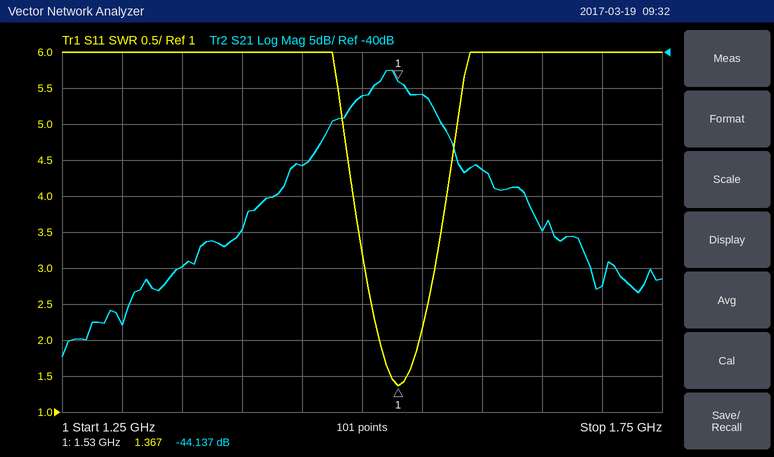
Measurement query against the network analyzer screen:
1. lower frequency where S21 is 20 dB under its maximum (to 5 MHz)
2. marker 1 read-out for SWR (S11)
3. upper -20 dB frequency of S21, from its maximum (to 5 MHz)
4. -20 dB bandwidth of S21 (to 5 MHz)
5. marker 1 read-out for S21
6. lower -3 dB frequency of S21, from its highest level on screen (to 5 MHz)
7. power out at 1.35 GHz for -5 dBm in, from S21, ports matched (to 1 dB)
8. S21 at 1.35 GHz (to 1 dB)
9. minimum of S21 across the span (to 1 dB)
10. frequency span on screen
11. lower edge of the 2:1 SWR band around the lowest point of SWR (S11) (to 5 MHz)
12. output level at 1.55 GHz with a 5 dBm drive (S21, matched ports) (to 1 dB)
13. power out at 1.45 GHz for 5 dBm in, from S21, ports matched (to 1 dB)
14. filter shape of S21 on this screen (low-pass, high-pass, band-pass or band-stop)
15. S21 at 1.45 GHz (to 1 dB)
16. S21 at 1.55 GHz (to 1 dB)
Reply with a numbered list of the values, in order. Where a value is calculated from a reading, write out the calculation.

1. 1.405 GHz
2. 1.367
3. 1.645 GHz
4. 1.645 GHz − 1.405 GHz = 240 MHz
5. -44.137 dB
6. 1.505 GHz
7. -5 dBm + (-70 dB) = -75 dBm
8. -70 dB
9. -82 dB
10. 500 MHz
11. 1.515 GHz
12. 5 dBm + (-46 dB) = -41 dBm
13. 5 dBm + (-56 dB) = -51 dBm
14. band-pass
15. -56 dB
16. -46 dB
